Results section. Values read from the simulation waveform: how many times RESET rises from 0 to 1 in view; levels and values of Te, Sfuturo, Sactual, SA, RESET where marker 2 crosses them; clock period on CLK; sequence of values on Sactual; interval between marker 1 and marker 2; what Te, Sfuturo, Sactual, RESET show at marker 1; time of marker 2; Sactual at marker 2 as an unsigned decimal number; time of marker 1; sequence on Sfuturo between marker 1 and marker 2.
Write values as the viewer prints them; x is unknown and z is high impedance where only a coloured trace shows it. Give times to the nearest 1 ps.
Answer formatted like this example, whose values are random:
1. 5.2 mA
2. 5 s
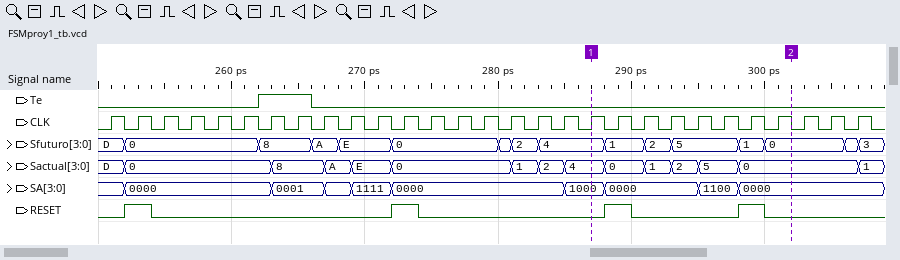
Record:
1. 4
2. Te=0, Sfuturo=0, Sactual=0, SA=0000, RESET=0
3. 2 ps
4. D, 0, 8, A, E, 0, 1, 2, 4, 0, 1, 2, 5, 0, 1
5. 15 ps
6. Te=0, Sfuturo=4, Sactual=4, RESET=0
7. 302 ps
8. 0
9. 287 ps
10. 4, 1, 2, 5, 1, 0
